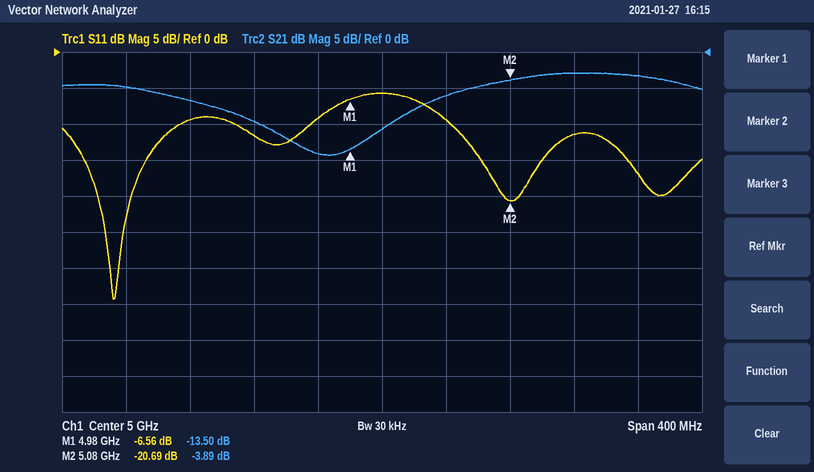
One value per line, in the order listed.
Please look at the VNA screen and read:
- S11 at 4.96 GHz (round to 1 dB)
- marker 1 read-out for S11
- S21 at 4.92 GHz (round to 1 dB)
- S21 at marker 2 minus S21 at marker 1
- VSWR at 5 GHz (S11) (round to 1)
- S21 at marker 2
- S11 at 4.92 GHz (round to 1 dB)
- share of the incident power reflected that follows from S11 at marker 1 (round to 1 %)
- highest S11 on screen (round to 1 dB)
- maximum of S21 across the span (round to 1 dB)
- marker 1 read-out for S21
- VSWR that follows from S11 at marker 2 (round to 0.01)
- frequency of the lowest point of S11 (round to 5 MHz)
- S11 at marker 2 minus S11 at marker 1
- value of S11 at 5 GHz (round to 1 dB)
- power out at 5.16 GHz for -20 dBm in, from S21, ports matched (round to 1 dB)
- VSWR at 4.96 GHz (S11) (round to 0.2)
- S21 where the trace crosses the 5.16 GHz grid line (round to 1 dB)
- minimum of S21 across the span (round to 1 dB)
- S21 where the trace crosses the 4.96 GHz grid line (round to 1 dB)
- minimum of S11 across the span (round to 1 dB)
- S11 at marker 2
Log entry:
-9 dB
-6.56 dB
-10 dB
9.61 dB
3
-3.89 dB
-12 dB
22 %
-6 dB
-3 dB
-13.50 dB
1.20
4.830 GHz
-14.13 dB
-6 dB
-23 dBm
2.0
-3 dB
-14 dB
-14 dB
-34 dB
-20.69 dB
